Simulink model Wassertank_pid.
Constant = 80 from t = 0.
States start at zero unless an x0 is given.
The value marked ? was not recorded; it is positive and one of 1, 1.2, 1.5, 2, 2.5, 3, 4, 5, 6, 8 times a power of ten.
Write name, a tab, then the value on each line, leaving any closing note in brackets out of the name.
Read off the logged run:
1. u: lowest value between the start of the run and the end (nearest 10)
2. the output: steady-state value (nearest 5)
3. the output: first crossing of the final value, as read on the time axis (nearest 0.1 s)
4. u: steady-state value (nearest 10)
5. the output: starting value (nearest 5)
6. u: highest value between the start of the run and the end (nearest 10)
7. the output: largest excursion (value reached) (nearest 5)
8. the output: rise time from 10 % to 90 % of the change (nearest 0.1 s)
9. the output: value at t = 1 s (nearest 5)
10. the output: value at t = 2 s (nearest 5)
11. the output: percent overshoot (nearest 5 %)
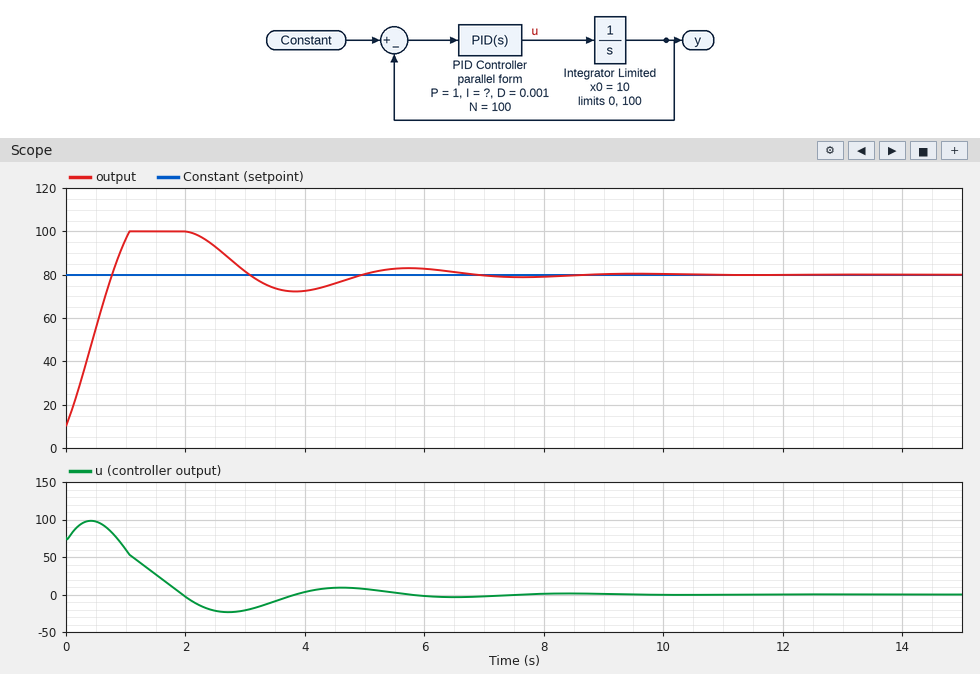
u: lowest value between the start of the run and the end	-20
the output: steady-state value	80
the output: first crossing of the final value, as read on the time axis	0.8 s
u: steady-state value	0
the output: starting value	10
u: highest value between the start of the run and the end	100
the output: largest excursion (value reached)	100
the output: rise time from 10 % to 90 % of the change	0.6 s
the output: value at t = 1 s	95
the output: value at t = 2 s	100
the output: percent overshoot	30 %
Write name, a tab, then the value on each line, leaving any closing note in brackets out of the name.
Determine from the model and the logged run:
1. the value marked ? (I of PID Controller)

the value marked ?	3
